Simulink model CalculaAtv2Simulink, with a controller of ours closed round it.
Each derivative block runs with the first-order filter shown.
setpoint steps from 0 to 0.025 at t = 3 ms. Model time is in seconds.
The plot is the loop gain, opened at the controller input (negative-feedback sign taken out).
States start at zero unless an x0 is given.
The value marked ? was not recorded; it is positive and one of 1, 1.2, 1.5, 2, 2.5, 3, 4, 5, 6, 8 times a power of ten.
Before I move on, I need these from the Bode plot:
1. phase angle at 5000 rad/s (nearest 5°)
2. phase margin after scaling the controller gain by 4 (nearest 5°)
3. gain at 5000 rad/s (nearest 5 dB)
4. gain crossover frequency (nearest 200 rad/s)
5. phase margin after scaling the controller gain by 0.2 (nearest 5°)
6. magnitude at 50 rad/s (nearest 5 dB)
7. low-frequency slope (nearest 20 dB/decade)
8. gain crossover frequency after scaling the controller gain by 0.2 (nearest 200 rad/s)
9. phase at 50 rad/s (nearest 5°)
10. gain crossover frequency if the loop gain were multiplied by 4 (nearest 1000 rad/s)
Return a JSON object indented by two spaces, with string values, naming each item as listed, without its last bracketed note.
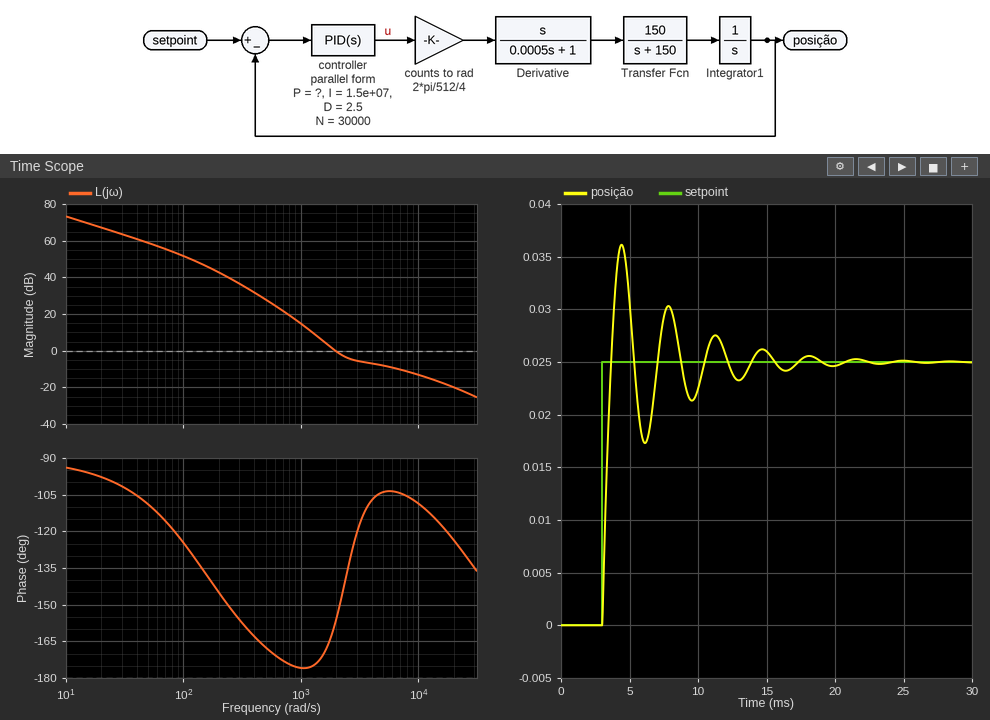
{
  "phase angle at 5000 rad/s": "-105°",
  "phase margin after scaling the controller gain by 4": "75°",
  "gain at 5000 rad/s": "-10 dB",
  "gain crossover frequency": "2000 rad/s",
  "phase margin after scaling the controller gain by 0.2": "5°",
  "magnitude at 50 rad/s": "60 dB",
  "low-frequency slope": "-20 dB/decade",
  "gain crossover frequency after scaling the controller gain by 0.2": "1000 rad/s",
  "phase at 50 rad/s": "-110°",
  "gain crossover frequency if the loop gain were multiplied by 4": "9000 rad/s"
}
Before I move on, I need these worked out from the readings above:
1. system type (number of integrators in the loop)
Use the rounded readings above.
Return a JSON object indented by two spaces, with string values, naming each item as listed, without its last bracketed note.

{
  "system type": "1"
}
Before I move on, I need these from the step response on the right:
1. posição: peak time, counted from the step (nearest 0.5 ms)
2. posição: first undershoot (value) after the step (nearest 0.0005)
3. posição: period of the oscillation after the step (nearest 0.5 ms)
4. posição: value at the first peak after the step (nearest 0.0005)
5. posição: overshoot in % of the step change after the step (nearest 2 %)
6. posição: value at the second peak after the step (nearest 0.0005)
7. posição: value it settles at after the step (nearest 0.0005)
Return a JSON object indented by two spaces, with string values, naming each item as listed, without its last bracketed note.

{
  "posição: peak time, counted from the step": "1.5 ms",
  "posição: first undershoot (value) after the step": "0.0175",
  "posição: period of the oscillation after the step": "3.5 ms",
  "posição: value at the first peak after the step": "0.0360",
  "posição: overshoot in % of the step change after the step": "44 %",
  "posição: value at the second peak after the step": "0.0305",
  "posição: value it settles at after the step": "0.0250"
}
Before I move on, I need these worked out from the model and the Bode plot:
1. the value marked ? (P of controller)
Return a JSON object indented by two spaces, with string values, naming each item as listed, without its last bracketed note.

{
  "the value marked ?": "5000"
}
